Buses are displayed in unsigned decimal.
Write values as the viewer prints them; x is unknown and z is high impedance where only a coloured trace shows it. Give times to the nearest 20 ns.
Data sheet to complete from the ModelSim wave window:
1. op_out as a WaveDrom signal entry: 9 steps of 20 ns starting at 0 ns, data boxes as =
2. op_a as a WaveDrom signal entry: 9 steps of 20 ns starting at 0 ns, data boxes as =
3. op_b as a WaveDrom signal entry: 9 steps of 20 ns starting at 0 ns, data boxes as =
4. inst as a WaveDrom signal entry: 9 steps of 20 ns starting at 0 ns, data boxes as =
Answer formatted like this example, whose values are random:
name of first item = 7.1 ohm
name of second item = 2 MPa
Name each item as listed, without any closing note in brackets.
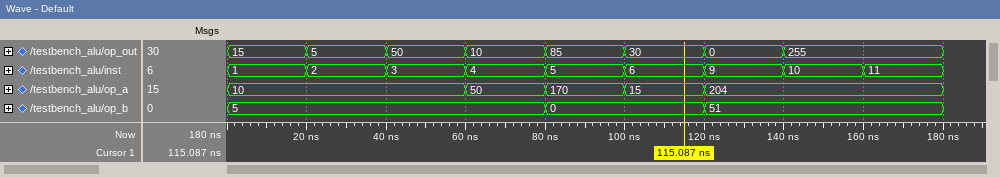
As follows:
op_out as a WaveDrom signal entry: 9 steps of 20 ns starting at 0 ns, data boxes as = = {name: 'op_out', wave: '========.', data: '15 5 50 10 85 30 0 255'}
op_a as a WaveDrom signal entry: 9 steps of 20 ns starting at 0 ns, data boxes as = = {name: 'op_a', wave: '=..====..', data: '10 50 170 15 204'}
op_b as a WaveDrom signal entry: 9 steps of 20 ns starting at 0 ns, data boxes as = = {name: 'op_b', wave: '=...=.=..', data: '5 0 51'}
inst as a WaveDrom signal entry: 9 steps of 20 ns starting at 0 ns, data boxes as = = {name: 'inst', wave: '=========', data: '1 2 3 4 5 6 9 10 11'}
